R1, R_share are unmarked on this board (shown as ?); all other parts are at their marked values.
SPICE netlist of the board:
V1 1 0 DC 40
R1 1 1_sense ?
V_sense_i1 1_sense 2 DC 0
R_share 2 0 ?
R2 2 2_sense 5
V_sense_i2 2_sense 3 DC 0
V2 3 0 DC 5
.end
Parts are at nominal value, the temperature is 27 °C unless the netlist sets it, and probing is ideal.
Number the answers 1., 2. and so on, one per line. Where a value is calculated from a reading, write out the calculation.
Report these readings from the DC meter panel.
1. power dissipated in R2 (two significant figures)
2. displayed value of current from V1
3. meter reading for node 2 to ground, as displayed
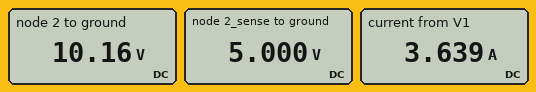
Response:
1. (10.16 V - 5 V)^2 / 5 Ω = 5.3 W
2. 3.639 A
3. 10.16 V
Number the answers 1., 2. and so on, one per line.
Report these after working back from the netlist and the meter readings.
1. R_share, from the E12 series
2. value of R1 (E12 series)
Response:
1. 3.9 Ω
2. 8.2 Ω
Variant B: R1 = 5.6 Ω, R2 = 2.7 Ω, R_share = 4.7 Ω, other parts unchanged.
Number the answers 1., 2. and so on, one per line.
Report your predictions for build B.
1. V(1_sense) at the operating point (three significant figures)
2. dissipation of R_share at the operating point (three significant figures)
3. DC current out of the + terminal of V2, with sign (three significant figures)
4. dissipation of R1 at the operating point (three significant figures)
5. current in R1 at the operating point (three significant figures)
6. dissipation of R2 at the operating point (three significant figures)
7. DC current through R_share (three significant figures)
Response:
1. 11.8 V
2. 29.7 W
3. -2.52 A
4. 142 W
5. 5.03 A
6. 17.2 W
7. 2.51 A
